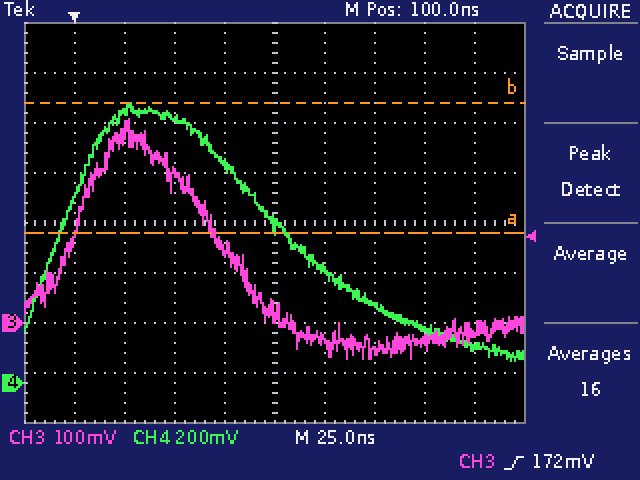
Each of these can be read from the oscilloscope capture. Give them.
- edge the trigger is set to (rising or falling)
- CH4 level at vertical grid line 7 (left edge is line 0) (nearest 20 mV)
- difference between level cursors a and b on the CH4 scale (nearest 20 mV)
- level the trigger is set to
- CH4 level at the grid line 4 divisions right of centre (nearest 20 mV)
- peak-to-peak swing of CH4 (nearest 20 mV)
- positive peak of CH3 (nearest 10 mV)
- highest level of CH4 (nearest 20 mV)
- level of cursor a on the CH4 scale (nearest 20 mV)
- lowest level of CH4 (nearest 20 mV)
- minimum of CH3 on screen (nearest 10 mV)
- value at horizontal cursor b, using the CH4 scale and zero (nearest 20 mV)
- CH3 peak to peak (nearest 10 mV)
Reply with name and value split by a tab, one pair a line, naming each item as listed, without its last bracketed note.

edge the trigger is set to	rising
CH4 level at vertical grid line 7 (left edge is line 0)	320 mV
difference between level cursors a and b on the CH4 scale	520 mV
level the trigger is set to	172 mV
CH4 level at the grid line 4 divisions right of centre	140 mV
peak-to-peak swing of CH4	1.04 V
positive peak of CH3	410 mV
highest level of CH4	1.12 V
level of cursor a on the CH4 scale	600 mV
lowest level of CH4	80 mV
minimum of CH3 on screen	-70 mV
value at horizontal cursor b, using the CH4 scale and zero	1.12 V
CH3 peak to peak	480 mV
